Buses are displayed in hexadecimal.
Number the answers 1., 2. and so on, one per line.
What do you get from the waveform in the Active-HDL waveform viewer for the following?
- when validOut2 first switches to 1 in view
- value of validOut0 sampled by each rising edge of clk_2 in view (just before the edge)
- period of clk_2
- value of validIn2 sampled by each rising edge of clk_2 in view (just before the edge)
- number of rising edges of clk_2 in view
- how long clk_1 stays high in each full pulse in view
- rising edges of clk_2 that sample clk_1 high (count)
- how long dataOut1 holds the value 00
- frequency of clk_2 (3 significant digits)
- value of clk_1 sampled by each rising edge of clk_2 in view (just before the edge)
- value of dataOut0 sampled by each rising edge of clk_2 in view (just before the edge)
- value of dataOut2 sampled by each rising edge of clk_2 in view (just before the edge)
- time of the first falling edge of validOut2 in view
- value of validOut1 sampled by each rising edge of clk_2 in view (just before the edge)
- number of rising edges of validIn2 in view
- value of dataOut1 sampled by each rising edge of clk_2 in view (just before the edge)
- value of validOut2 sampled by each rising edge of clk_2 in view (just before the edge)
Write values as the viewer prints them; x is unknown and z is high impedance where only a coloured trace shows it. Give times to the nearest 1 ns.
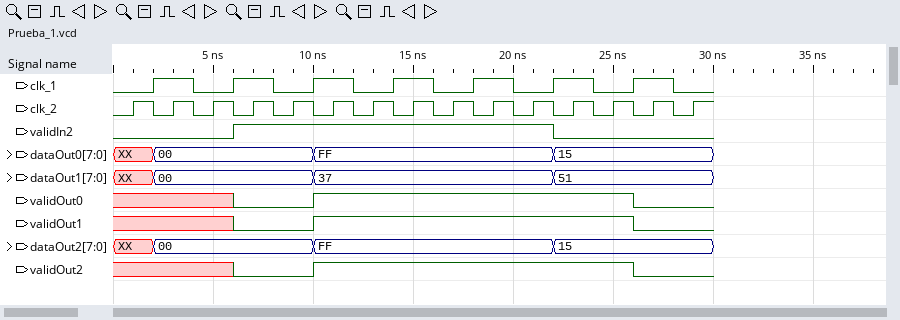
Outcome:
1. 10 ns
2. x x x 0 0 1 1 1 1 1 1 1 1 0 0
3. 2 ns
4. 0 0 0 1 1 1 1 1 1 1 1 0 0 0 0
5. 15
6. 2 ns, 2 ns, 2 ns, 2 ns, 2 ns, 2 ns, 2 ns
7. 7
8. 8 ns
9. 500 MHz
10. 0 1 0 1 0 1 0 1 0 1 0 1 0 1 0
11. XX, 00, 00, 00, 00, FF, FF, FF, FF, FF, FF, 15, 15, 15, 15
12. XX, 00, 00, 00, 00, FF, FF, FF, FF, FF, FF, 15, 15, 15, 15
13. 26 ns
14. x x x 0 0 1 1 1 1 1 1 1 1 0 0
15. 1
16. XX, 00, 00, 00, 00, 37, 37, 37, 37, 37, 37, 51, 51, 51, 51
17. x x x 0 0 1 1 1 1 1 1 1 1 0 0
